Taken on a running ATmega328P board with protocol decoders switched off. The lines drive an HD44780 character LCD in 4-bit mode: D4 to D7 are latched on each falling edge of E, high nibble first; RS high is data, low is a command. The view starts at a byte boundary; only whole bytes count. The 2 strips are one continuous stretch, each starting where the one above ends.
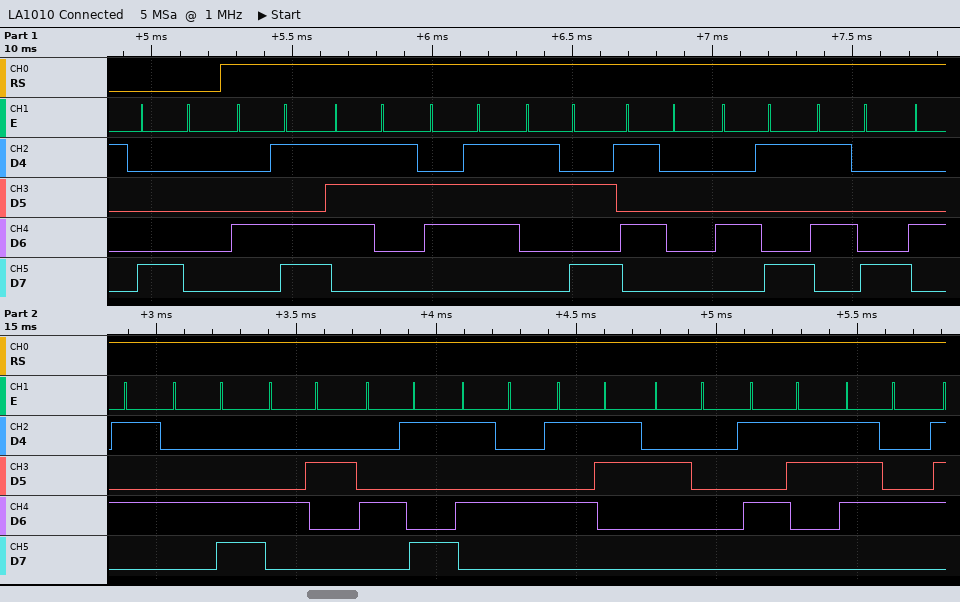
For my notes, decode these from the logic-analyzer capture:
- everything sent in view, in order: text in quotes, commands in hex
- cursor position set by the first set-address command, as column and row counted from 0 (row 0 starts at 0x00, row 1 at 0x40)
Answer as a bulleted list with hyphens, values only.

- 0x80 "Msg:PIXELBITS St"
- column 0, row 0
